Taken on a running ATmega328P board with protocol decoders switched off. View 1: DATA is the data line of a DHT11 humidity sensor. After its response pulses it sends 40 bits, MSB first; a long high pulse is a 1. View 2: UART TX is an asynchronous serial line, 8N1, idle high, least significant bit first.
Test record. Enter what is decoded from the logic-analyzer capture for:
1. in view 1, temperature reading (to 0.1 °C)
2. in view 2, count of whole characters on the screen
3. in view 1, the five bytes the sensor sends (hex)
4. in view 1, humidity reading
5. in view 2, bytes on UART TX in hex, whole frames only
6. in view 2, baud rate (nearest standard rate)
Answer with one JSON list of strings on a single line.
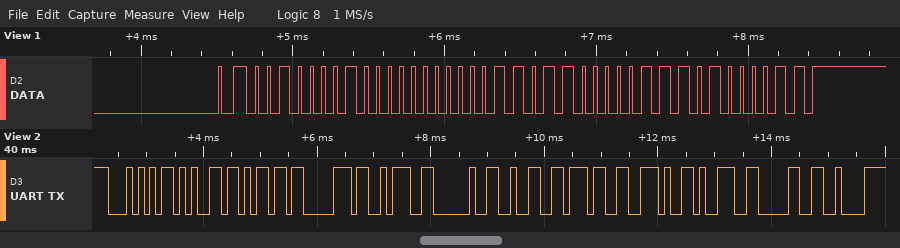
["27.7 °C", "12", "21 00 1B 07 43", "33 %", "0x54 0x65 0x6D 0x70 0x3A 0x20 0x32 0x37 0x2E 0x39 0x30 0xC2", "9600 baud"]
